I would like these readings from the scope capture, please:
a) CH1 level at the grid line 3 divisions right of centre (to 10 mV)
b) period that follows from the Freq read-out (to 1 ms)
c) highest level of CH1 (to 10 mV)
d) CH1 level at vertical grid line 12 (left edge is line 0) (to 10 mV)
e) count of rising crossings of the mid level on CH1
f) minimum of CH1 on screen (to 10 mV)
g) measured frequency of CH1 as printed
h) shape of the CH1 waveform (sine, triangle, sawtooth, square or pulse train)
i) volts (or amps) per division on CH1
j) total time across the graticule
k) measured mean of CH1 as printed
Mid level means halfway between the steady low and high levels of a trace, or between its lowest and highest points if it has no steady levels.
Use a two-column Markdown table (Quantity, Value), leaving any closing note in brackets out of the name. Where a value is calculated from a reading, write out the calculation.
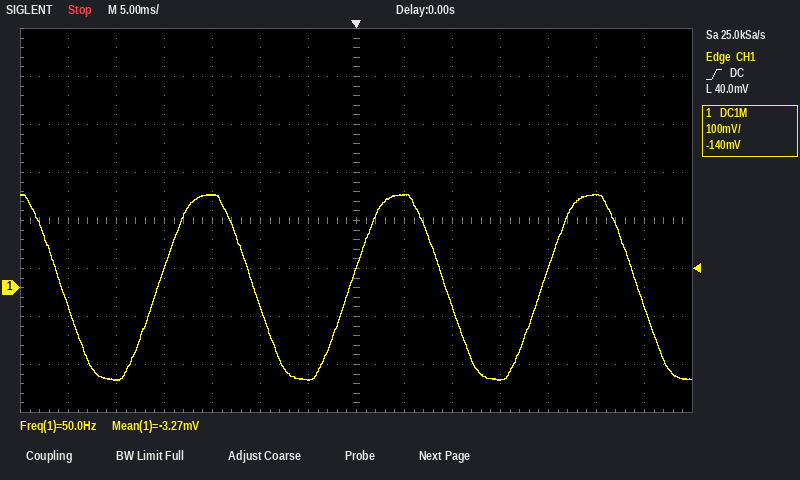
| Quantity | Value |
|---|---|
| CH1 level at the grid line 3 divisions right of centre | -190 mV |
| period that follows from the Freq read-out | 1 / 50.0 Hz ≈ 20 ms |
| highest level of CH1 | 190 mV |
| CH1 level at vertical grid line 12 (left edge is line 0) | 190 mV |
| count of rising crossings of the mid level on CH1 | 3 |
| minimum of CH1 on screen | -190 mV |
| measured frequency of CH1 as printed | 50.0 Hz |
| shape of the CH1 waveform | sine |
| volts (or amps) per division on CH1 | 100 mV |
| total time across the graticule | 70 ms |
| measured mean of CH1 as printed | -3.27 mV |
